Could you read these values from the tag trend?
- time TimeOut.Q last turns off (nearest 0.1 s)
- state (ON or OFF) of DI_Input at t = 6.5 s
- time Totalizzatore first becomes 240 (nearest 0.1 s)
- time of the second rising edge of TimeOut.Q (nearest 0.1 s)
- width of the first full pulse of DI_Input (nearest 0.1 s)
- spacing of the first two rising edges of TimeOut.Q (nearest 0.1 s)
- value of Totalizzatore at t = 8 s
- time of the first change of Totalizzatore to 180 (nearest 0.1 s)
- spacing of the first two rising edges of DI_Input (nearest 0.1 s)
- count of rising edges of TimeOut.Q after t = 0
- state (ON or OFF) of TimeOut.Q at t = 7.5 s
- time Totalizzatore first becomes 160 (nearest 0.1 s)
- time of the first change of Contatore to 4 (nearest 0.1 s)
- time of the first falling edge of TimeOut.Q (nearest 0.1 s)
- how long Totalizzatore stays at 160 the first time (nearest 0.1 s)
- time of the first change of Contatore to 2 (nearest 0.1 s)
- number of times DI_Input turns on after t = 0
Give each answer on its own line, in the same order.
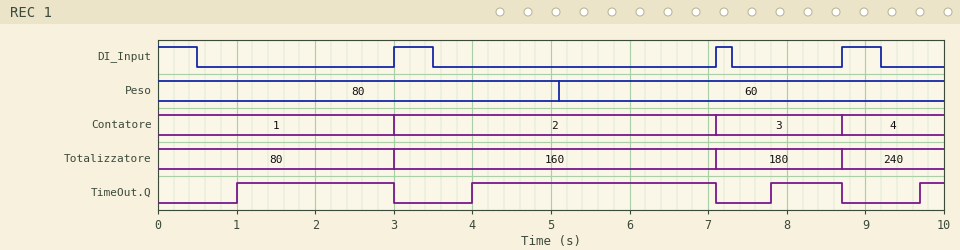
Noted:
8.7 s
OFF
8.7 s
4.0 s
0.5 s
3.0 s
180
7.1 s
4.1 s
4
OFF
3.0 s
8.7 s
3.0 s
4.1 s
3.0 s
3
